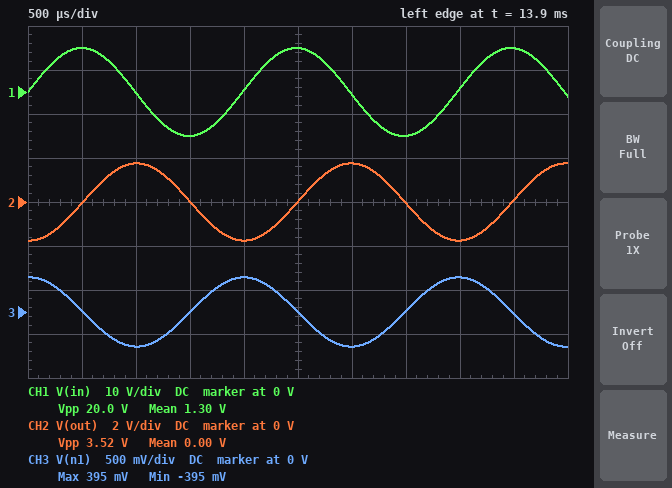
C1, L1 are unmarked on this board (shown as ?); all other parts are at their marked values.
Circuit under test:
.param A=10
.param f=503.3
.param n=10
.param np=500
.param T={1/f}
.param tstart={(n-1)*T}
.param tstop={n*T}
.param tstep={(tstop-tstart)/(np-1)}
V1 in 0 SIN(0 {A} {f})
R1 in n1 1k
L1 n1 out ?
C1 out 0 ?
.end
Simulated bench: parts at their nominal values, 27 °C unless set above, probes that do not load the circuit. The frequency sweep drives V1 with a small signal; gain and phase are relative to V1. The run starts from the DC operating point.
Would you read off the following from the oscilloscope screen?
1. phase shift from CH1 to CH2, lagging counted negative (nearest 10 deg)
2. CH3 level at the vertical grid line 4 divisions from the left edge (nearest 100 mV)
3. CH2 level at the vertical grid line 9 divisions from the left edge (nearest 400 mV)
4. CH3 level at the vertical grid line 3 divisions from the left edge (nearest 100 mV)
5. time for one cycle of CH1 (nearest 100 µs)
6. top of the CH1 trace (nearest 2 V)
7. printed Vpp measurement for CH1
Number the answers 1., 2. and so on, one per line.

1. -90 deg
2. 400 mV
3. 0 V
4. 0 V
5. 2.0 ms
6. 10 V
7. 20.0 V
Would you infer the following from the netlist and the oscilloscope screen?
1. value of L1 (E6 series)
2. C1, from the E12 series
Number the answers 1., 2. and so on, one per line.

1. 68 mH
2. 1.8 µF
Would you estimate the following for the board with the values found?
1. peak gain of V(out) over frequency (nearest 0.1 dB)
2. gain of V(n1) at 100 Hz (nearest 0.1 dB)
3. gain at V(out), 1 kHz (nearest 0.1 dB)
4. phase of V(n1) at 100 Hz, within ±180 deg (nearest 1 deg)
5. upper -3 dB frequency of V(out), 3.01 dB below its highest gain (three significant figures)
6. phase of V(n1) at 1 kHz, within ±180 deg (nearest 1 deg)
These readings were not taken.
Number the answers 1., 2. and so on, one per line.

1. 0 dB
2. -3.8 dB
3. -21.5 dB
4. -50 deg
5. 91.9 Hz
6. 71 deg
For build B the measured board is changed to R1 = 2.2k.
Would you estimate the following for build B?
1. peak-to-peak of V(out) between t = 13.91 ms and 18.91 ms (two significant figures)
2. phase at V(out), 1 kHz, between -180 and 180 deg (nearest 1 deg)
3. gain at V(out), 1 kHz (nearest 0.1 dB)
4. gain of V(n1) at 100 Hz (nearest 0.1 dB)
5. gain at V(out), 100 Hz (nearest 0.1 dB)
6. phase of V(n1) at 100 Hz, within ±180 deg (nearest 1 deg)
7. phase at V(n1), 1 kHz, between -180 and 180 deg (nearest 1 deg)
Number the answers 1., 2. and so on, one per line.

1. 1.6 V
2. -99 deg
3. -28.0 dB
4. -8.9 dB
5. -8.5 dB
6. -69 deg
7. 81 deg
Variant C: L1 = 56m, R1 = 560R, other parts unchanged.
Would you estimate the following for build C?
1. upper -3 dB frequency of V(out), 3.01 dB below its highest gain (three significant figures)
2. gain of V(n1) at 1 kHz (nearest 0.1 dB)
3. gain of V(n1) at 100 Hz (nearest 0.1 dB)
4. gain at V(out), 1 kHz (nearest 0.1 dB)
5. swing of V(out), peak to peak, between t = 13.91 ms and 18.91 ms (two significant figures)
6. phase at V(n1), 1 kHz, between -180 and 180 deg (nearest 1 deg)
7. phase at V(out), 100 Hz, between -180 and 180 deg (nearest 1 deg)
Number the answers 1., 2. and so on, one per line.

1. 175 Hz
2. -7.4 dB
3. -1.6 dB
4. -16.9 dB
5. 6.3 V
6. 65 deg
7. -33 deg
